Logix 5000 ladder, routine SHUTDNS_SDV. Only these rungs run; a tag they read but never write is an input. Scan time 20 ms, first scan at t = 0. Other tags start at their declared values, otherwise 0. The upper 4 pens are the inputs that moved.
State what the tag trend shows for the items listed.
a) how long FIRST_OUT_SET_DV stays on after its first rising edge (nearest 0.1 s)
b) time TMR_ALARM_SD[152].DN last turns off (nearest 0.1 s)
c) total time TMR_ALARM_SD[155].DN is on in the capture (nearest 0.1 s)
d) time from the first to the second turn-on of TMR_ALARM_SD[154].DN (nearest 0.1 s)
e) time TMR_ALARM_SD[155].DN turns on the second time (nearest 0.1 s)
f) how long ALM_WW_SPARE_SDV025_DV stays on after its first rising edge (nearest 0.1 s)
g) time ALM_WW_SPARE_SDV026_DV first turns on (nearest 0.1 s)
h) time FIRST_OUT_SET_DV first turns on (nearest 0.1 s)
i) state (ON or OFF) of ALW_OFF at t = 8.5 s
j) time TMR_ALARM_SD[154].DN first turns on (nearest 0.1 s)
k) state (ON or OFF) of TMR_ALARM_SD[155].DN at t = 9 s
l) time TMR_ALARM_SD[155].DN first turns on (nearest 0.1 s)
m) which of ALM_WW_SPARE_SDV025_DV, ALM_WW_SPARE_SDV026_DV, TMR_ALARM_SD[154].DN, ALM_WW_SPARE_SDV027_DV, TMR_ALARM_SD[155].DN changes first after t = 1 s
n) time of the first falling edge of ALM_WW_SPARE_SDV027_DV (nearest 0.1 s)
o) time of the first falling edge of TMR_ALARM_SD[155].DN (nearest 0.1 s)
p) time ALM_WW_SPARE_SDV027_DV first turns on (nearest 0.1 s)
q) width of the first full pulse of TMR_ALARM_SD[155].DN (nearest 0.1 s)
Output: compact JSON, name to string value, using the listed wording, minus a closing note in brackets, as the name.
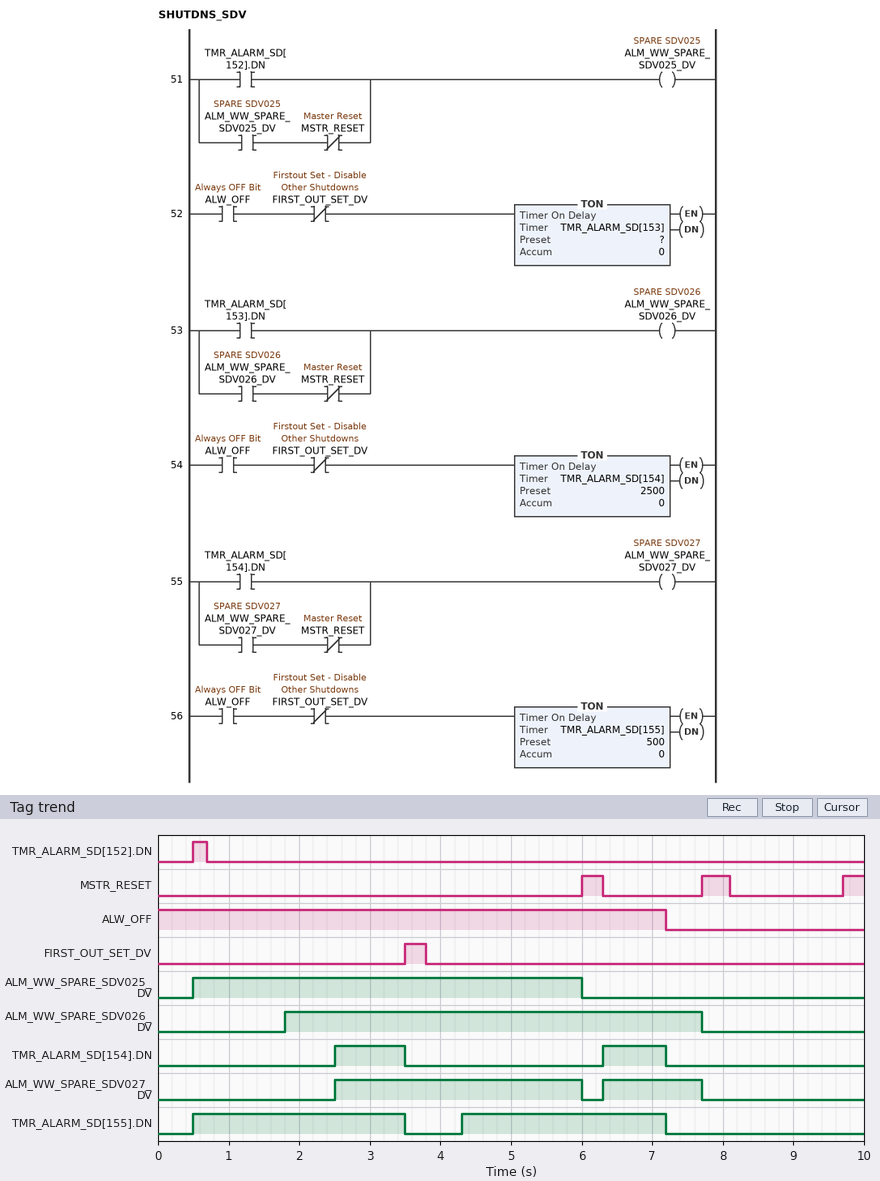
{"how long FIRST_OUT_SET_DV stays on after its first rising edge": "0.3 s", "time TMR_ALARM_SD[152].DN last turns off": "0.7 s", "total time TMR_ALARM_SD[155].DN is on in the capture": "5.9 s", "time from the first to the second turn-on of TMR_ALARM_SD[154].DN": "3.8 s", "time TMR_ALARM_SD[155].DN turns on the second time": "4.3 s", "how long ALM_WW_SPARE_SDV025_DV stays on after its first rising edge": "5.5 s", "time ALM_WW_SPARE_SDV026_DV first turns on": "1.8 s", "time FIRST_OUT_SET_DV first turns on": "3.5 s", "state (ON or OFF) of ALW_OFF at t = 8.5 s": "OFF", "time TMR_ALARM_SD[154].DN first turns on": "2.5 s", "state (ON or OFF) of TMR_ALARM_SD[155].DN at t = 9 s": "OFF", "time TMR_ALARM_SD[155].DN first turns on": "0.5 s", "which of ALM_WW_SPARE_SDV025_DV, ALM_WW_SPARE_SDV026_DV, TMR_ALARM_SD[154].DN, ALM_WW_SPARE_SDV027_DV, TMR_ALARM_SD[155].DN changes first after t = 1 s": "ALM_WW_SPARE_SDV026_DV", "time of the first falling edge of ALM_WW_SPARE_SDV027_DV": "6.0 s", "time of the first falling edge of TMR_ALARM_SD[155].DN": "3.5 s", "time ALM_WW_SPARE_SDV027_DV first turns on": "2.5 s", "width of the first full pulse of TMR_ALARM_SD[155].DN": "3.0 s"}
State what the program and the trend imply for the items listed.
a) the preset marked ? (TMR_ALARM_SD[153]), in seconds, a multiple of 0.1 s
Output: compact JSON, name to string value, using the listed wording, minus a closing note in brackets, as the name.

{"the preset marked ? (TMR_ALARM_SD[153]), in seconds, a multiple of 0.1 s": "1.8 s"}
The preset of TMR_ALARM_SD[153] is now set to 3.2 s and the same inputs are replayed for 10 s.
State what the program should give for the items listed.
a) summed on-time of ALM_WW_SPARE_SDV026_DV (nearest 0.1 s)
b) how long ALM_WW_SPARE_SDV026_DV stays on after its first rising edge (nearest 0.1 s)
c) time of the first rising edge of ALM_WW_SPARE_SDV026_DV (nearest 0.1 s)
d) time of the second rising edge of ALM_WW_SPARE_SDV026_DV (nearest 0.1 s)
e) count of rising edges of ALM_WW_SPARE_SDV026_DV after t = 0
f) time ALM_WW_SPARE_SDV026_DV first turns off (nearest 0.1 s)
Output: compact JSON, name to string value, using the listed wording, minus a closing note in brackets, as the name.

{"summed on-time of ALM_WW_SPARE_SDV026_DV": "3.5 s", "how long ALM_WW_SPARE_SDV026_DV stays on after its first rising edge": "2.8 s", "time of the first rising edge of ALM_WW_SPARE_SDV026_DV": "3.2 s", "time of the second rising edge of ALM_WW_SPARE_SDV026_DV": "7.0 s", "count of rising edges of ALM_WW_SPARE_SDV026_DV after t = 0": "2", "time ALM_WW_SPARE_SDV026_DV first turns off": "6.0 s"}
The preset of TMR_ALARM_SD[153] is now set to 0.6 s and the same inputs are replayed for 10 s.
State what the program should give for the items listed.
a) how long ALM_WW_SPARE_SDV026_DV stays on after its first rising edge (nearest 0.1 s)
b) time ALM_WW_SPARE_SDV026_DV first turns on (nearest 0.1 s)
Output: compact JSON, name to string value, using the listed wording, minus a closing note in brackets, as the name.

{"how long ALM_WW_SPARE_SDV026_DV stays on after its first rising edge": "7.1 s", "time ALM_WW_SPARE_SDV026_DV first turns on": "0.6 s"}
